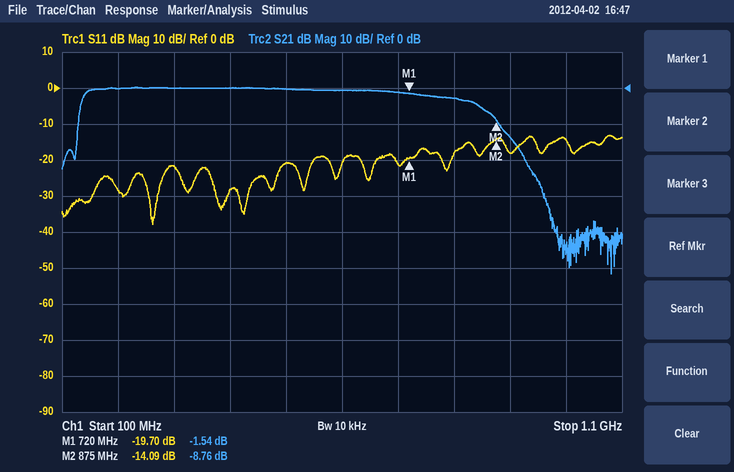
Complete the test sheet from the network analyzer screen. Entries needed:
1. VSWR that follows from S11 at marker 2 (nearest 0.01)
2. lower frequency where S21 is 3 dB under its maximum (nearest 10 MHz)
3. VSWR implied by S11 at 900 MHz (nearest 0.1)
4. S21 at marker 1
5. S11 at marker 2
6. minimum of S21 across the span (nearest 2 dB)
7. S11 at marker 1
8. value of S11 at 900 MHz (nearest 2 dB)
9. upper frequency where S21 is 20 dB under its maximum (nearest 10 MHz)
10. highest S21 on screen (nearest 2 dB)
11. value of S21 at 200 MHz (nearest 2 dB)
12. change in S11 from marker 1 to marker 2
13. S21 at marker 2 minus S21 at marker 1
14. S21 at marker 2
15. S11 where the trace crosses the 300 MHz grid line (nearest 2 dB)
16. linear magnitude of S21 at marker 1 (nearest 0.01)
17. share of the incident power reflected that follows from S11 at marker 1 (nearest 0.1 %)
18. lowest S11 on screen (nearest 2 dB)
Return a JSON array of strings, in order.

["1.49", "140 MHz", "1.3", "-1.54 dB", "-14.09 dB", "-52 dB", "-19.70 dB", "-18 dB", "930 MHz", "0 dB", "0 dB", "5.61 dB", "-7.22 dB", "-8.76 dB", "-22 dB", "0.84", "1.1 %", "-38 dB"]
